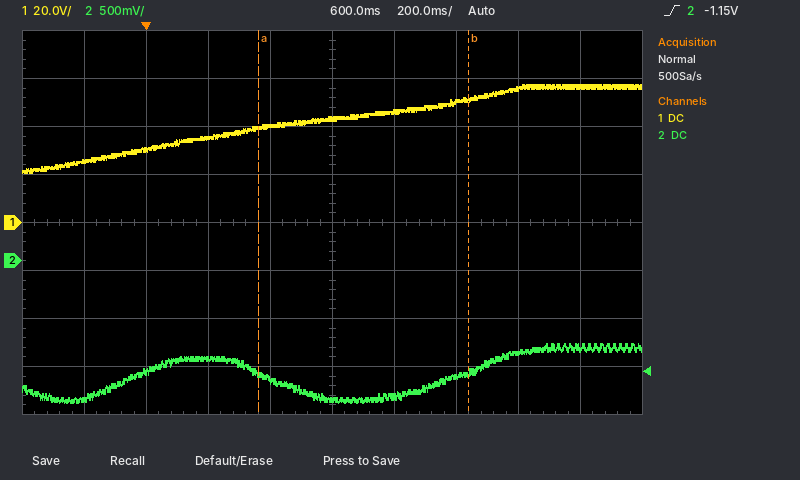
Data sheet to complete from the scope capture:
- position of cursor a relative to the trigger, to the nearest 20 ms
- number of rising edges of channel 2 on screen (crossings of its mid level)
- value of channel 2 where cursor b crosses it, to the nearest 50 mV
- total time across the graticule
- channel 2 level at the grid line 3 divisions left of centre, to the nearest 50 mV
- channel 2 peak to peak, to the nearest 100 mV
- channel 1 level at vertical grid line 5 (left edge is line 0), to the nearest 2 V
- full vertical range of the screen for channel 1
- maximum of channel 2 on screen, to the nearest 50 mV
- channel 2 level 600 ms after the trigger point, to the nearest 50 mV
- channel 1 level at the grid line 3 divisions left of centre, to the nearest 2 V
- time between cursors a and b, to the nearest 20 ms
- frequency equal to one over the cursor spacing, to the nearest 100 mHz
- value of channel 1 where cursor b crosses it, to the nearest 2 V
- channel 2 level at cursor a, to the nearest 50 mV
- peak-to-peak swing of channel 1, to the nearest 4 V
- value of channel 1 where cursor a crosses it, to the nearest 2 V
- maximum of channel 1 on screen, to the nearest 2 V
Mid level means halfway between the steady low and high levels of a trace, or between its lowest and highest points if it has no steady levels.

+360 ms
2
-1.15 V
2 s
-1.15 V
600 mV
44 V
160 V
-850 mV
-1.45 V
30 V
680 ms
1.5 Hz
52 V
-1.15 V
36 V
40 V
58 V
